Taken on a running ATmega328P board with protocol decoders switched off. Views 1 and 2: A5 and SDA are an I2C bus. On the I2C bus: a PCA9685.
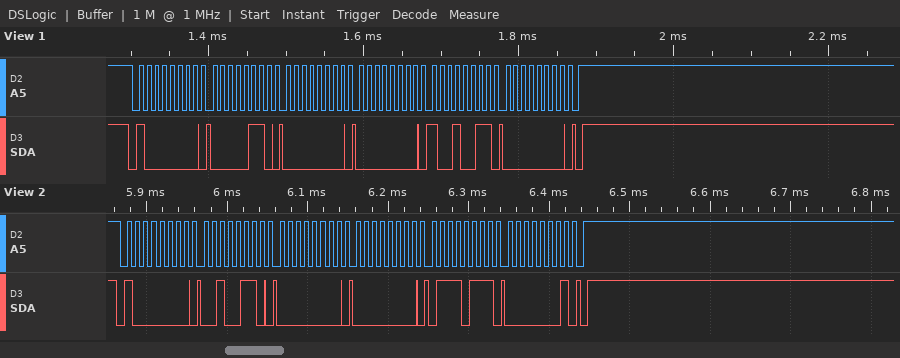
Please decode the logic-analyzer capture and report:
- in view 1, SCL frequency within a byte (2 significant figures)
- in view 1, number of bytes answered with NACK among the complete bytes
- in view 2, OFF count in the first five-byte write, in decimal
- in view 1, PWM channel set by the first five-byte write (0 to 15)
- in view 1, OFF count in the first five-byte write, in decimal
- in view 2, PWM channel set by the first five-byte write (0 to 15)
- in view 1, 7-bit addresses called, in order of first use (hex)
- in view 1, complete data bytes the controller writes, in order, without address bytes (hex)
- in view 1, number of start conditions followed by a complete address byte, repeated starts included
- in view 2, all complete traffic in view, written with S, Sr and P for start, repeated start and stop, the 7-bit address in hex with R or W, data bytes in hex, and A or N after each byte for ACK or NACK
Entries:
100 kHz
0
375
0
147
8
0x40
06 00 00 93 00
1
S 40W A 26 A 00 A 00 A 77 A 01 A P
